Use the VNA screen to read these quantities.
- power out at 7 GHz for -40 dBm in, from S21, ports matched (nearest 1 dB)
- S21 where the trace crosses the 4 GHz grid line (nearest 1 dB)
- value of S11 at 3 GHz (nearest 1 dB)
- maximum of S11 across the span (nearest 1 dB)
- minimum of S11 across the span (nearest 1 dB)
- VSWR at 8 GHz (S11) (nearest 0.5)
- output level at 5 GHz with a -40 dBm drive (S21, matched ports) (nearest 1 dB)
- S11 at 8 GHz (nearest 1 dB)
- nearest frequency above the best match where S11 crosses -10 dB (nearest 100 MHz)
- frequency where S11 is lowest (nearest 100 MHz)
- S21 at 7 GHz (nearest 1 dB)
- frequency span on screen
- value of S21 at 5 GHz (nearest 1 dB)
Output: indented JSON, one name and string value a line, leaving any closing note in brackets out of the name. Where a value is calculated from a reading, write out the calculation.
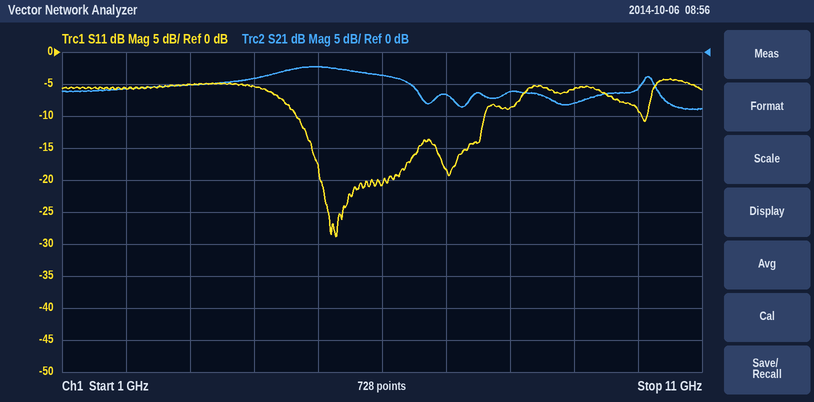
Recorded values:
{
  "power out at 7 GHz for -40 dBm in, from S21, ports matched": "-40 dBm + (-7 dB) = -47 dBm",
  "S21 where the trace crosses the 4 GHz grid line": "-4 dB",
  "value of S11 at 3 GHz": "-5 dB",
  "maximum of S11 across the span": "-4 dB",
  "minimum of S11 across the span": "-29 dB",
  "VSWR at 8 GHz (S11)": "|Γ| = 10^(-9/20) = 0.3548; VSWR = (1 + 0.3548)/(1 − 0.3548) ≈ 2.10, so 2.0 to the nearest 0.5",
  "output level at 5 GHz with a -40 dBm drive (S21, matched ports)": "-40 dBm + (-2 dB) = -42 dBm",
  "S11 at 8 GHz": "-9 dB",
  "nearest frequency above the best match where S11 crosses -10 dB": "7.6 GHz",
  "frequency where S11 is lowest": "5.3 GHz",
  "S21 at 7 GHz": "-7 dB",
  "frequency span on screen": "10 GHz",
  "value of S21 at 5 GHz": "-2 dB"
}
